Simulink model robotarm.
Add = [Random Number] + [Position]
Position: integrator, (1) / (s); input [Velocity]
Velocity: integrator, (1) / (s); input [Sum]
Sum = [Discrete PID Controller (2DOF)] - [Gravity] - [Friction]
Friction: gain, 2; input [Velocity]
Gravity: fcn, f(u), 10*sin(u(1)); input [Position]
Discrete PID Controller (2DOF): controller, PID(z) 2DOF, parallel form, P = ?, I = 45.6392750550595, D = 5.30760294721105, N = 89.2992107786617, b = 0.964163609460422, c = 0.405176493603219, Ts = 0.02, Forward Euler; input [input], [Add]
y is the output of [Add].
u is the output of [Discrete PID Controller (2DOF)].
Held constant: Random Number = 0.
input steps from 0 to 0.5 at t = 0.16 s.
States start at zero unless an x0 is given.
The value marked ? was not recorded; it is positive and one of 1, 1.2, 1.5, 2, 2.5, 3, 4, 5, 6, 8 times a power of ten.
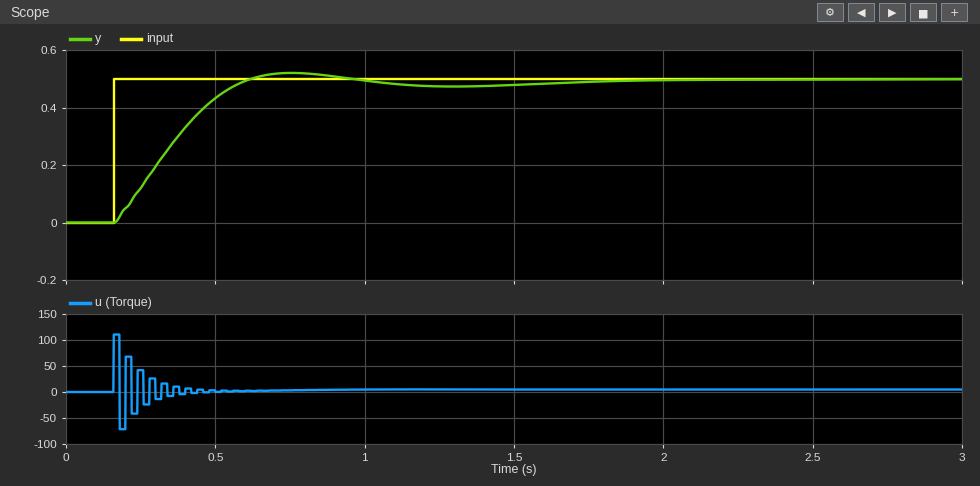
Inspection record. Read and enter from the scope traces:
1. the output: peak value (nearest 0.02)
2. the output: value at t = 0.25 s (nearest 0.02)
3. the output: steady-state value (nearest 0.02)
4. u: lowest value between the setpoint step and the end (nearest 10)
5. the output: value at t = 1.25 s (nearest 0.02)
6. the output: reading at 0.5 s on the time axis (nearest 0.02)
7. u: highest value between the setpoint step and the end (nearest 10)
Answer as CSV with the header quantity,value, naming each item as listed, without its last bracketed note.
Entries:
quantity,value
the output: peak value,0.52
the output: value at t = 0.25 s,0.12
the output: steady-state value,0.50
u: lowest value between the setpoint step and the end,-70
the output: value at t = 1.25 s,0.48
the output: reading at 0.5 s on the time axis,0.44
u: highest value between the setpoint step and the end,110
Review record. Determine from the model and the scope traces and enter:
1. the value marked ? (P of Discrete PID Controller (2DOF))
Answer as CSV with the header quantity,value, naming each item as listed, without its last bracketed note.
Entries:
quantity,value
the value marked ? (P of Discrete PID Controller (2DOF)),30
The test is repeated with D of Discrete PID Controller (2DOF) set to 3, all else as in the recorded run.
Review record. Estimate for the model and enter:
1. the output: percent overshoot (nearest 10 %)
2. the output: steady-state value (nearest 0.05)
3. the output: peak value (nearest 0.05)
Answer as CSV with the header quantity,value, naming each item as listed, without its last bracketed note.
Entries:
quantity,value
the output: percent overshoot,20 %
the output: steady-state value,0.50
the output: peak value,0.60
